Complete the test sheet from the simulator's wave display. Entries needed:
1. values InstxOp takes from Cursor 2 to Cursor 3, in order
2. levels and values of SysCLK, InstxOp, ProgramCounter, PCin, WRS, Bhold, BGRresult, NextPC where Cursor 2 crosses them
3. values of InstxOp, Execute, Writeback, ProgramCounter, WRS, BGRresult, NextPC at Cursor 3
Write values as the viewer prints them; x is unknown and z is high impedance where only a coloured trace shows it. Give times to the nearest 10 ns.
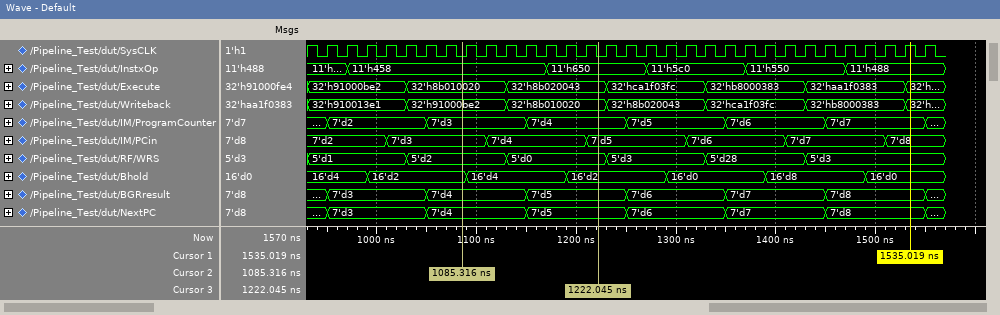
11'h458, 11'h650
SysCLK=0, InstxOp=11'h458, ProgramCounter=7'd3, PCin=7'd3, WRS=5'd2, Bhold=16'd2, BGRresult=7'd4, NextPC=7'd4
InstxOp=11'h650, Execute=32'h8b020043, Writeback=32'h8b010020, ProgramCounter=7'd4, WRS=5'd0, BGRresult=7'd5, NextPC=7'd5
